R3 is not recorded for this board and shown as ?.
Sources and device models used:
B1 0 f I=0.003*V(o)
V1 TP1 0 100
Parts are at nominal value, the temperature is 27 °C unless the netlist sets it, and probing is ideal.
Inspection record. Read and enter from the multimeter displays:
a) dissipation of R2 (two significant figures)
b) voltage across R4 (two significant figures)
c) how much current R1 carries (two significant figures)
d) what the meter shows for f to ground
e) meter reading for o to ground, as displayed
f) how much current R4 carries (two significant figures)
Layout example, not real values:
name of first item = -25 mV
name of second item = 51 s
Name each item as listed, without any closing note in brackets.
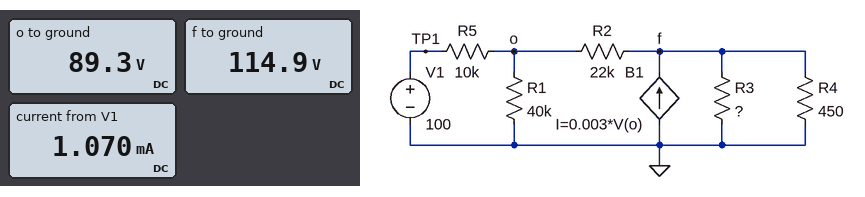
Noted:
dissipation of R2 = 30 mW
voltage across R4 = 110 V
how much current R1 carries = 2.2 mA
what the meter shows for f to ground = 114.9 V
meter reading for o to ground, as displayed = 89.3 V
how much current R4 carries = 260 mA
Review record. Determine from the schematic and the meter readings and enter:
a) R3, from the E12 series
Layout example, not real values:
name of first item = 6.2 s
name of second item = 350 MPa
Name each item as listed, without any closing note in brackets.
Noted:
R3, from the E12 series = 10 kΩ
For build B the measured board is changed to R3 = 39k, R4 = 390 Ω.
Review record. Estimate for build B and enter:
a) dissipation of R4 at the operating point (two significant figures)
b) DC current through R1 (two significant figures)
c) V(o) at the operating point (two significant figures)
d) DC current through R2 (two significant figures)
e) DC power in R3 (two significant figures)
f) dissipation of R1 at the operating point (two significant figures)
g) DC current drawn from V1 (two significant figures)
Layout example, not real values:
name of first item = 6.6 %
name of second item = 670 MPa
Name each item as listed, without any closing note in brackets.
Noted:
dissipation of R4 at the operating point = 25 W
DC current through R1 = 2.1 mA
V(o) at the operating point = 85 V
DC current through R2 = 600 µA
DC power in R3 = 250 mW
dissipation of R1 at the operating point = 180 mW
DC current drawn from V1 = 1.5 mA
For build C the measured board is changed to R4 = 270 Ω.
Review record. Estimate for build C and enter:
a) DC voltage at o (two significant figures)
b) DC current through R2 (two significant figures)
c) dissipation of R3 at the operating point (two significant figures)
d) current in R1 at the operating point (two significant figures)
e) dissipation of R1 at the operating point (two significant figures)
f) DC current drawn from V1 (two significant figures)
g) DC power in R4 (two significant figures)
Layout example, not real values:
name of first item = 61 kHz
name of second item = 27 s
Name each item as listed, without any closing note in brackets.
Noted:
DC voltage at o = 74 V
DC current through R2 = 710 µA
dissipation of R3 at the operating point = 350 mW
current in R1 at the operating point = 1.9 mA
dissipation of R1 at the operating point = 140 mW
DC current drawn from V1 = 2.6 mA
DC power in R4 = 13 W
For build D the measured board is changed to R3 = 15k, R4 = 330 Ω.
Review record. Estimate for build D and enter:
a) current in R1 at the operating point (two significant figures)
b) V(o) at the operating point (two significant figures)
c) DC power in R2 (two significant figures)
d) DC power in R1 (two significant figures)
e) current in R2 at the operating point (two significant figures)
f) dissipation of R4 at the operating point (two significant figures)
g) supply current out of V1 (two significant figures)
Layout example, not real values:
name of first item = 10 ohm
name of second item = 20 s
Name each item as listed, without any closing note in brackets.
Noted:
current in R1 at the operating point = 2.0 mA
V(o) at the operating point = 79 V
DC power in R2 = 270 µW
DC power in R1 = 160 mW
current in R2 at the operating point = 110 µA
dissipation of R4 at the operating point = 18 W
supply current out of V1 = 2.1 mA
